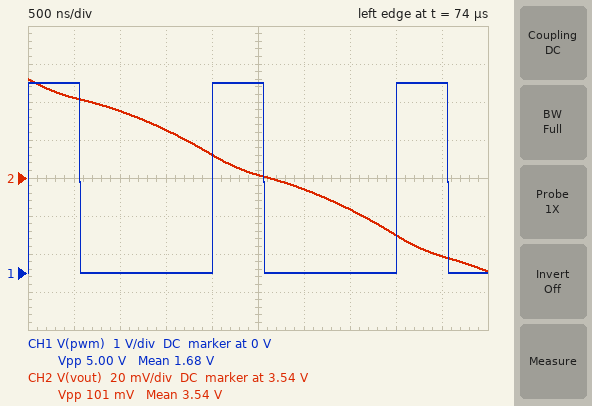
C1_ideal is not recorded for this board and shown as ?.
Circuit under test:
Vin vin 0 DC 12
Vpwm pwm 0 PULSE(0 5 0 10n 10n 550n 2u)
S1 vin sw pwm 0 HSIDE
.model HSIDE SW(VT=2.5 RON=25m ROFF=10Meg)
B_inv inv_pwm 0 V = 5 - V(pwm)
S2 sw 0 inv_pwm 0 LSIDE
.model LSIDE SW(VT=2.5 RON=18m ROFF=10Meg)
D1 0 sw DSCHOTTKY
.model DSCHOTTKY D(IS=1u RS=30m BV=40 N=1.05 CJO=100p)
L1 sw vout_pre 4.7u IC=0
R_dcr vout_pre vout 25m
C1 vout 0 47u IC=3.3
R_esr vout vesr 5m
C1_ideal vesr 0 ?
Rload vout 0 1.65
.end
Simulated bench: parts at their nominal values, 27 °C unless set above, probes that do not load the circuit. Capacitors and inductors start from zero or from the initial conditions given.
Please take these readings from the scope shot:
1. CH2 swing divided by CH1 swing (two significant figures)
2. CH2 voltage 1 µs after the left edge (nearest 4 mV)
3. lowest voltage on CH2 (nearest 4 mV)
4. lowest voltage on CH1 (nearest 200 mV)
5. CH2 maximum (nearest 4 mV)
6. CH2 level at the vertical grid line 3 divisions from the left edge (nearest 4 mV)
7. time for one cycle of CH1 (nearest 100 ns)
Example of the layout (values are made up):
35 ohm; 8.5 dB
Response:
0.020; 3.576 V; 3.492 V; 0 V; 3.592 V; 3.564 V; 2.0 µs
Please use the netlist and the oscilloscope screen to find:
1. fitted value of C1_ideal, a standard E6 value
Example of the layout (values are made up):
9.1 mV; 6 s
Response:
15 µF
